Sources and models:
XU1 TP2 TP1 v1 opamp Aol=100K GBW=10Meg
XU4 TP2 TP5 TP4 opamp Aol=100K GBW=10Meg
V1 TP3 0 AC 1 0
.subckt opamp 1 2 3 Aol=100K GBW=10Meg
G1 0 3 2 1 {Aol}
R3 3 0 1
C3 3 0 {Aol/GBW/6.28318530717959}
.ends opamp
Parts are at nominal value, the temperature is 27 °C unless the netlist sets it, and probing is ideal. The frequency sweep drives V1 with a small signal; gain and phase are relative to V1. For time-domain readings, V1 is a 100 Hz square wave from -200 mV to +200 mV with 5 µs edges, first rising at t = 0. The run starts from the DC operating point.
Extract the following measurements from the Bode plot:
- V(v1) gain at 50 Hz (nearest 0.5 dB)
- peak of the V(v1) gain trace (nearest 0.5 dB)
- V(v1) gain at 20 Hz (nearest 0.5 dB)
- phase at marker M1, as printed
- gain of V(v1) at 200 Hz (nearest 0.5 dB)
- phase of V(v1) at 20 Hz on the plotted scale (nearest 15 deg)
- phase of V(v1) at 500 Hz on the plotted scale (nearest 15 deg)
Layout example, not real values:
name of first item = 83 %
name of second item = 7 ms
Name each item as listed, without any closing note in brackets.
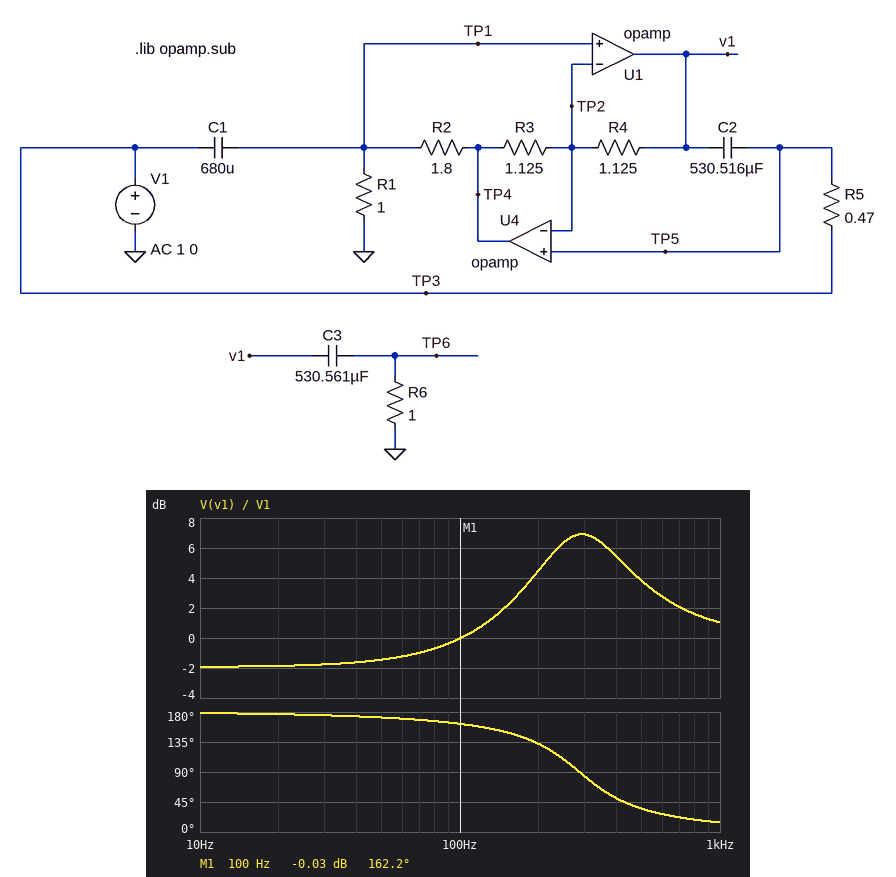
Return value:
V(v1) gain at 50 Hz = -1.5 dB
peak of the V(v1) gain trace = 7.0 dB
V(v1) gain at 20 Hz = -2.0 dB
phase at marker M1, as printed = 162.2 deg
gain of V(v1) at 200 Hz = 4.5 dB
phase of V(v1) at 20 Hz on the plotted scale = 180 deg
phase of V(v1) at 500 Hz on the plotted scale = 30 deg
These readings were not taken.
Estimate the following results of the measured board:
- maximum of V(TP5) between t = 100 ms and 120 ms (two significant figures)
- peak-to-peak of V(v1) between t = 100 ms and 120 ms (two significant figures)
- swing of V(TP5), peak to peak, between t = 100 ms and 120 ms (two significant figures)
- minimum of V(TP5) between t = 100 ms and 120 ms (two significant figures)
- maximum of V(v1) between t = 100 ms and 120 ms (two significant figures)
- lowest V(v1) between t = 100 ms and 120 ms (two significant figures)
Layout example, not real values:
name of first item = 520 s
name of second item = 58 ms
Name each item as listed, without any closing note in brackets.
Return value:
maximum of V(TP5) between t = 100 ms and 120 ms = 250 mV
peak-to-peak of V(v1) between t = 100 ms and 120 ms = 1.1 V
swing of V(TP5), peak to peak, between t = 100 ms and 120 ms = 500 mV
minimum of V(TP5) between t = 100 ms and 120 ms = -250 mV
maximum of V(v1) between t = 100 ms and 120 ms = 570 mV
lowest V(v1) between t = 100 ms and 120 ms = -570 mV
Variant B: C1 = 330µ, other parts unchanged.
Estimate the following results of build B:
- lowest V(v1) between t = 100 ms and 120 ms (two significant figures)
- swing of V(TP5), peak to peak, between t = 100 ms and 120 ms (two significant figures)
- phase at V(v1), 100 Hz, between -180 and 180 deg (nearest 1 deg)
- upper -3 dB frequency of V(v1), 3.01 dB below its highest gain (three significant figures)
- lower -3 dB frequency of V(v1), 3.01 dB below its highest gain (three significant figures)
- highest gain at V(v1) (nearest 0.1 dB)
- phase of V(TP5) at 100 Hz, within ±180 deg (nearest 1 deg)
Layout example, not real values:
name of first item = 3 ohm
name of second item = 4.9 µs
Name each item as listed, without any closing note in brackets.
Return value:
lowest V(v1) between t = 100 ms and 120 ms = -560 mV
swing of V(TP5), peak to peak, between t = 100 ms and 120 ms = 450 mV
phase at V(v1), 100 Hz, between -180 and 180 deg = 163 deg
upper -3 dB frequency of V(v1), 3.01 dB below its highest gain = 1.41 kHz
lower -3 dB frequency of V(v1), 3.01 dB below its highest gain = 203 Hz
highest gain at V(v1) = 3.8 dB
phase of V(TP5) at 100 Hz, within ±180 deg = -17 deg
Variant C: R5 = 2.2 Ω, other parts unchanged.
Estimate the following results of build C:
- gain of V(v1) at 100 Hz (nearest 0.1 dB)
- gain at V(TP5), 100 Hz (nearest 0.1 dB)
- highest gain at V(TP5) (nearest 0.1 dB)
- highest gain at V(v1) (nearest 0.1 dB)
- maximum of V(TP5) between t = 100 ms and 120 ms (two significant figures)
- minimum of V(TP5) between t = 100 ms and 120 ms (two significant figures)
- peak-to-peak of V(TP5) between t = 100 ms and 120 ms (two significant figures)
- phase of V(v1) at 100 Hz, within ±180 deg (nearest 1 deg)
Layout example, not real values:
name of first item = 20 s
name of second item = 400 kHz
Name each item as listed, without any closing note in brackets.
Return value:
gain of V(v1) at 100 Hz = -0.2 dB
gain at V(TP5), 100 Hz = -10.1 dB
highest gain at V(TP5) = 0 dB
highest gain at V(v1) = 0.4 dB
maximum of V(TP5) between t = 100 ms and 120 ms = 230 mV
minimum of V(TP5) between t = 100 ms and 120 ms = -230 mV
peak-to-peak of V(TP5) between t = 100 ms and 120 ms = 470 mV
phase of V(v1) at 100 Hz, within ±180 deg = 108 deg
